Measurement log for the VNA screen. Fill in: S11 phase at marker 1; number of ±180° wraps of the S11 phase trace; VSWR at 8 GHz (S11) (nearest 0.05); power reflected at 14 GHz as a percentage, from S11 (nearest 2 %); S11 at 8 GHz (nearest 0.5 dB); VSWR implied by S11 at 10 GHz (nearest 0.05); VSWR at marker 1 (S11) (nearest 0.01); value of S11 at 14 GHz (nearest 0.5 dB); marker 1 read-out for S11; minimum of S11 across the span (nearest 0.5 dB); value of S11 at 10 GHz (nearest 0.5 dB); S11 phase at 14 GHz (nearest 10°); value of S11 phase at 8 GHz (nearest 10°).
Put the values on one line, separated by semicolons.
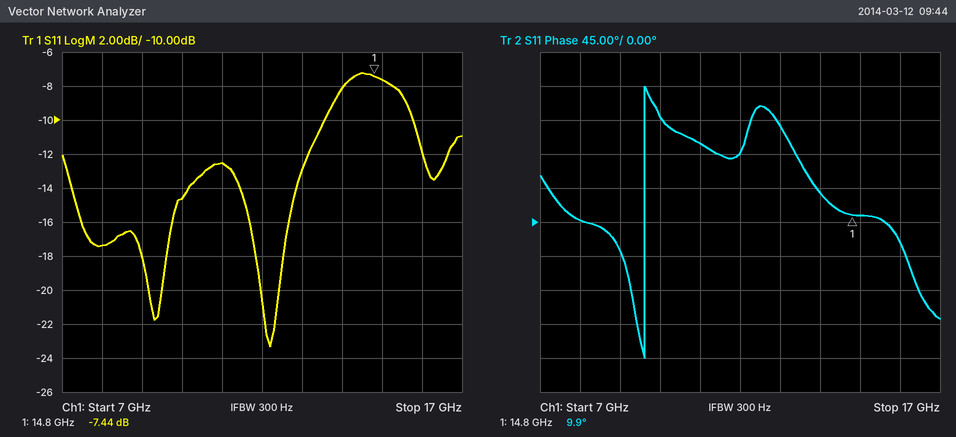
9.9°; 1; 1.30; 16 %; -17.5 dB; 1.45; 2.48; -8.0 dB; -7.44 dB; -23.5 dB; -14.5 dB; 40°; 0°
